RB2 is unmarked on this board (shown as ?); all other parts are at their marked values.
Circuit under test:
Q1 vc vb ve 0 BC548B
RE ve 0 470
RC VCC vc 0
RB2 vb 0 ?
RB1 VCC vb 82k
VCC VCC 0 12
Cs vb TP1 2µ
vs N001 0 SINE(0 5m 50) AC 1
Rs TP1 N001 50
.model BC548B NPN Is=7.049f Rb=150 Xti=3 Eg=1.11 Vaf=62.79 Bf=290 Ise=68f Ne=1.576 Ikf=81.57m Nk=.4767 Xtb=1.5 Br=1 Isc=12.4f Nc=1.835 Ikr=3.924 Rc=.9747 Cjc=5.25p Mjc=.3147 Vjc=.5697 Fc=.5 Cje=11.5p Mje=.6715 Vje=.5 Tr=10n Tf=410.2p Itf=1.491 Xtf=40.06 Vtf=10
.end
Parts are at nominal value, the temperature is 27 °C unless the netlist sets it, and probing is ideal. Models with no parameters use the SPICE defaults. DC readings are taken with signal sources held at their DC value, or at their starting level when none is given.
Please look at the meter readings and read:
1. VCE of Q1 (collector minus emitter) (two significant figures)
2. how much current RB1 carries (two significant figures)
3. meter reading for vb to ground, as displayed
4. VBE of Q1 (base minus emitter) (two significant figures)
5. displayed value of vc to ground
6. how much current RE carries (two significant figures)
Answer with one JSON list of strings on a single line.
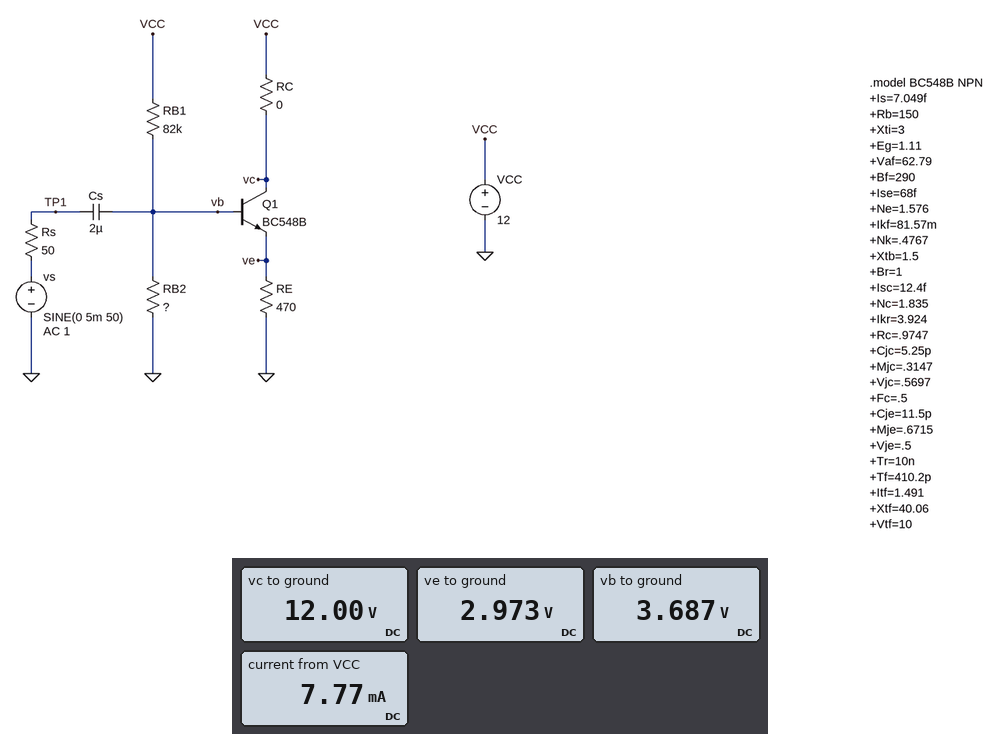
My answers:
["9.0 V", "100 µA", "3.687 V", "710 mV", "12.00 V", "6.3 mA"]
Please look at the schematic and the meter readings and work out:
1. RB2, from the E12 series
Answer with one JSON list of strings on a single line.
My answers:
["47 kΩ"]
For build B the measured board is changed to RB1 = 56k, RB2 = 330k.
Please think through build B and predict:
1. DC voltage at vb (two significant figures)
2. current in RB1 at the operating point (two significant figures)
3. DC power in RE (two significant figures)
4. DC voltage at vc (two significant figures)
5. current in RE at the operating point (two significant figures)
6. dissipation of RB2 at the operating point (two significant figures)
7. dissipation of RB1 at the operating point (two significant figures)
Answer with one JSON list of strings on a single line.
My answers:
["7.5 V", "80 µA", "97 mW", "12 V", "14 mA", "170 µW", "360 µW"]
